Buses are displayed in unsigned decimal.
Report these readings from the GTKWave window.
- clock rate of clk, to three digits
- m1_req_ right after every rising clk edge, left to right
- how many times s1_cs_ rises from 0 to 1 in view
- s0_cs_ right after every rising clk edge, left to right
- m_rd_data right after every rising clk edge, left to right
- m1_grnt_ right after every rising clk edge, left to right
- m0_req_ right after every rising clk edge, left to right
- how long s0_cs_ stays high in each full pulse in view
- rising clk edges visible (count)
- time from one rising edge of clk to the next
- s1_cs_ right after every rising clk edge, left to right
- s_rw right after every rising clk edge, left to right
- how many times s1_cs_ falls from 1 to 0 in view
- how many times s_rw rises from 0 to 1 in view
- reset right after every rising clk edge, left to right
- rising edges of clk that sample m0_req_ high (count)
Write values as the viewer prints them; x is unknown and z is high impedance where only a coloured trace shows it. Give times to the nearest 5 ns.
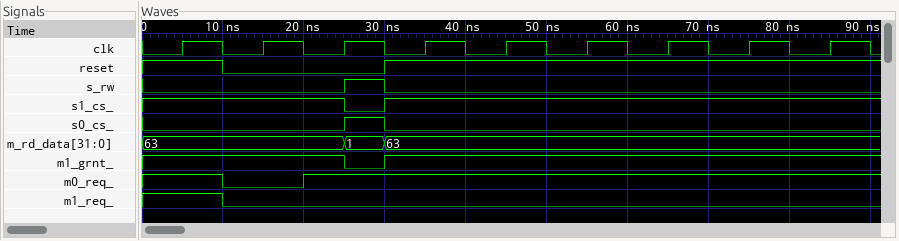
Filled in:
100 MHz
1 0 0 0 0 0 0 0 0
1
0 0 1 0 0 0 0 0 0
63, 63, 1, 63, 63, 63, 63, 63, 63
1 1 0 1 1 1 1 1 1
1 0 1 1 1 1 1 1 1
5 ns
9
10 ns
1 1 0 1 1 1 1 1 1
0 0 1 0 0 0 0 0 0
1
1
1 0 0 1 1 1 1 1 1
8
